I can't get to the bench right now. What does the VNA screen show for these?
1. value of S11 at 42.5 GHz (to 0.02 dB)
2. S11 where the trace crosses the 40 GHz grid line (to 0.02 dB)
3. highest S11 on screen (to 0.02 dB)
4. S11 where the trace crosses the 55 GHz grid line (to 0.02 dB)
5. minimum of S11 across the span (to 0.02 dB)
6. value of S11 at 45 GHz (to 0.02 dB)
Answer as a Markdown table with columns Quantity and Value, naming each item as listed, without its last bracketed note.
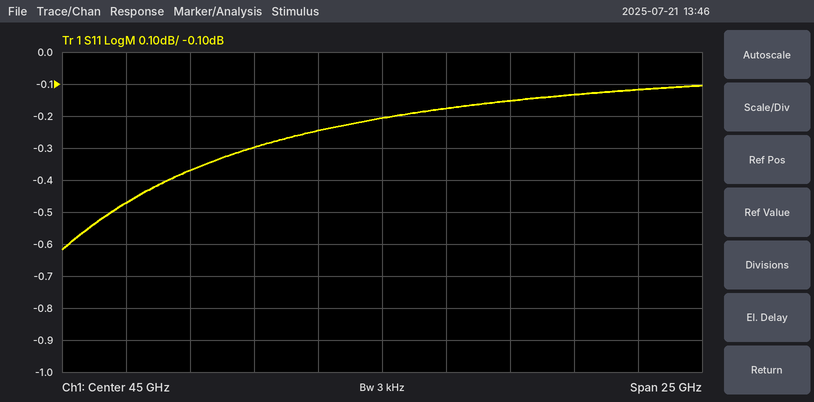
| Quantity | Value |
|---|---|
| value of S11 at 42.5 GHz | -0.24 dB |
| S11 where the trace crosses the 40 GHz grid line | -0.30 dB |
| highest S11 on screen | -0.10 dB |
| S11 where the trace crosses the 55 GHz grid line | -0.12 dB |
| minimum of S11 across the span | -0.62 dB |
| value of S11 at 45 GHz | -0.20 dB |
